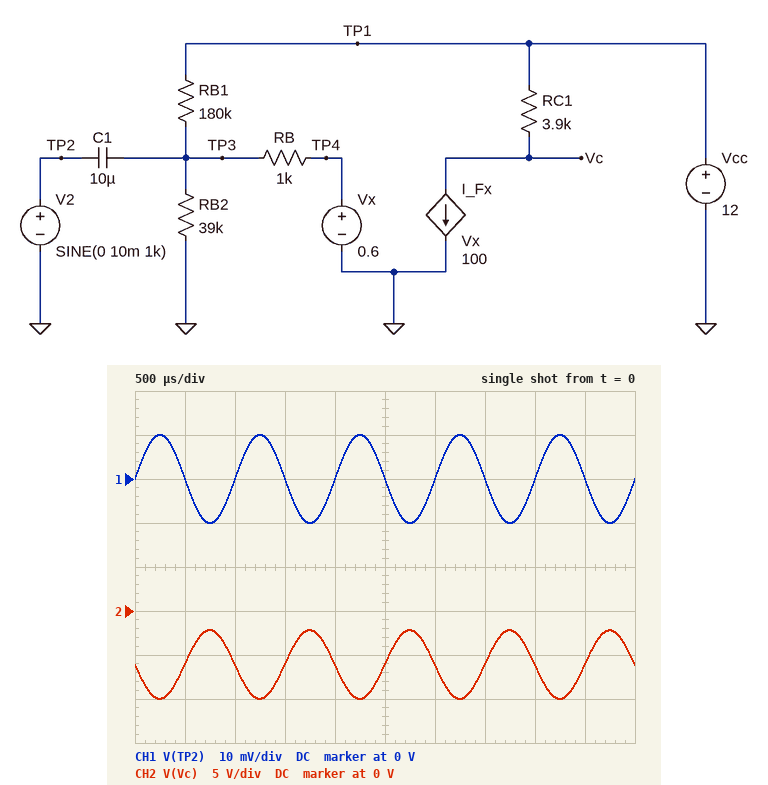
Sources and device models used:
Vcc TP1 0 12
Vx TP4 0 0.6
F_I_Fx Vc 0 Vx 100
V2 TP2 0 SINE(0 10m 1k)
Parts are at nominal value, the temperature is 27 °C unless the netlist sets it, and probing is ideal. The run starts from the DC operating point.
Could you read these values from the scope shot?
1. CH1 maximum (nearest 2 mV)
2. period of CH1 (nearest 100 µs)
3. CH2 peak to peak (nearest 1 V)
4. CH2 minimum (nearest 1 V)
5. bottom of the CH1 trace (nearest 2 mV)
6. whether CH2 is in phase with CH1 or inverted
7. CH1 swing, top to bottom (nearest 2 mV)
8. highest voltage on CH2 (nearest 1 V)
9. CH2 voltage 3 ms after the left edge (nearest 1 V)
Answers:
10 mV
1.0 ms
8 V
-10 V
-10 mV
inverted
20 mV
-2 V
-6 V
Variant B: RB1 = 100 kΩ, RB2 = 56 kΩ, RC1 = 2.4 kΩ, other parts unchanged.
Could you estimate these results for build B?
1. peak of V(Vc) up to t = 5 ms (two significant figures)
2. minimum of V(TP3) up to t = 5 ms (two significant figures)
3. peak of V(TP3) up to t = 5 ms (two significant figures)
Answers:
-9.7 V
690 mV
710 mV
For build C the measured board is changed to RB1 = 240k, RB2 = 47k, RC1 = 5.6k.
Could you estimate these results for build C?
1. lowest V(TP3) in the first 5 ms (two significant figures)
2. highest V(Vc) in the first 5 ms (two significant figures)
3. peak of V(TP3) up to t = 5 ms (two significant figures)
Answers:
620 mV
-1.3 V
640 mV
